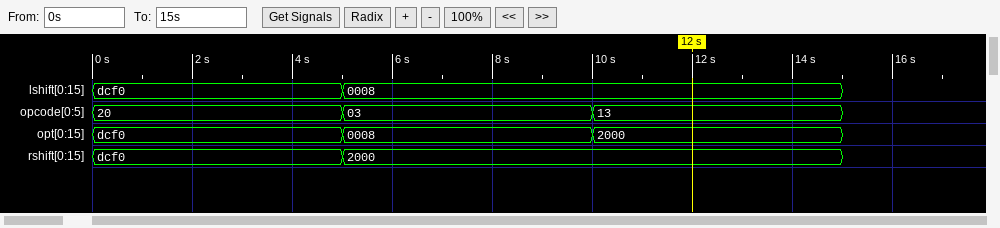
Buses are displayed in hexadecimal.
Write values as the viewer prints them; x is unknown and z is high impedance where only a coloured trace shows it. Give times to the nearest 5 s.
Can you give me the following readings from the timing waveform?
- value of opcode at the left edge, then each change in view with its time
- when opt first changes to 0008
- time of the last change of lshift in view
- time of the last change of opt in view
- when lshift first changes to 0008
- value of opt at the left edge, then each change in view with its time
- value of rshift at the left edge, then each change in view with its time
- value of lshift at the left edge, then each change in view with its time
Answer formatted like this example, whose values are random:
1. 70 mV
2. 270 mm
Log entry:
1. 20, 03 at 5 s, 13 at 10 s
2. 5 s
3. 5 s
4. 10 s
5. 5 s
6. dcf0, 0008 at 5 s, 2000 at 10 s
7. dcf0, 2000 at 5 s
8. dcf0, 0008 at 5 s
